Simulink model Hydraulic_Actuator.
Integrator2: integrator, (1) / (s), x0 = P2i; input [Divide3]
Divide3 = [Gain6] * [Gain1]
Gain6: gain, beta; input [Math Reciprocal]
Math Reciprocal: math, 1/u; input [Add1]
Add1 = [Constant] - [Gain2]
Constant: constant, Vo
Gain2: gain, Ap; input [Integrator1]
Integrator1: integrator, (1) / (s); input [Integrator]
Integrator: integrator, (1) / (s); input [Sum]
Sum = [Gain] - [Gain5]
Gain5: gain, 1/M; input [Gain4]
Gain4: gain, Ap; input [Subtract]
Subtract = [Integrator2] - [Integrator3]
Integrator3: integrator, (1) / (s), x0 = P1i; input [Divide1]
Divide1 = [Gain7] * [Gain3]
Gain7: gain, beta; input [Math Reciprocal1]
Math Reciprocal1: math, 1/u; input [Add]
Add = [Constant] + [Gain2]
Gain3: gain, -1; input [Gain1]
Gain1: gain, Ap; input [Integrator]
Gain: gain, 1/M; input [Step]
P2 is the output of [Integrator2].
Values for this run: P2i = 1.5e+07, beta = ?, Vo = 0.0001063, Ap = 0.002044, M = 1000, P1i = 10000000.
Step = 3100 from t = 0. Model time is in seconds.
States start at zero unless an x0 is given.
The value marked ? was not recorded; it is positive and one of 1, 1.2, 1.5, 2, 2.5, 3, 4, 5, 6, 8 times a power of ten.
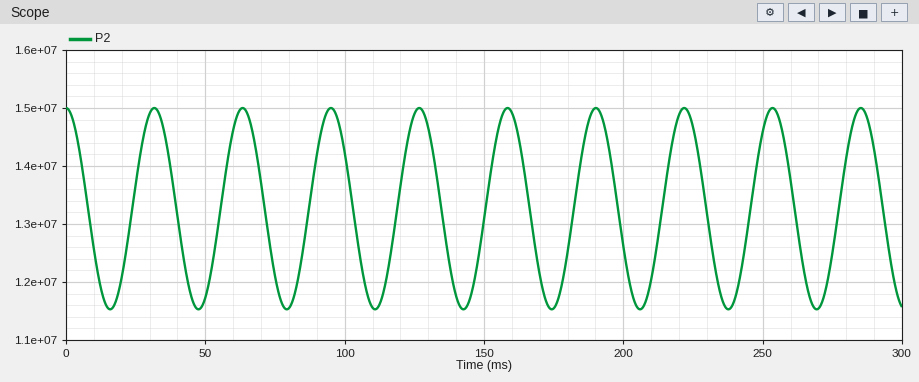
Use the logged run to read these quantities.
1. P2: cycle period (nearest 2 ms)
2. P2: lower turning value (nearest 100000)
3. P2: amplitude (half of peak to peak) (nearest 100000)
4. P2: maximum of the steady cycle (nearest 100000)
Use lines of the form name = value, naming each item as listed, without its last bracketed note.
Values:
P2: cycle period = 32 ms
P2: lower turning value = 11500000
P2: amplitude (half of peak to peak) = 1700000
P2: maximum of the steady cycle = 15000000
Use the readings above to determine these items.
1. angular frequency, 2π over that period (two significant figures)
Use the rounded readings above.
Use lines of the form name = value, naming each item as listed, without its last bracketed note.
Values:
angular frequency, 2π over that period = 0.20 rad/ms
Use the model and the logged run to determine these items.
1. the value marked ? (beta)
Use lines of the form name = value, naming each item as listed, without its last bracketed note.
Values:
the value marked ? = 5e+08
